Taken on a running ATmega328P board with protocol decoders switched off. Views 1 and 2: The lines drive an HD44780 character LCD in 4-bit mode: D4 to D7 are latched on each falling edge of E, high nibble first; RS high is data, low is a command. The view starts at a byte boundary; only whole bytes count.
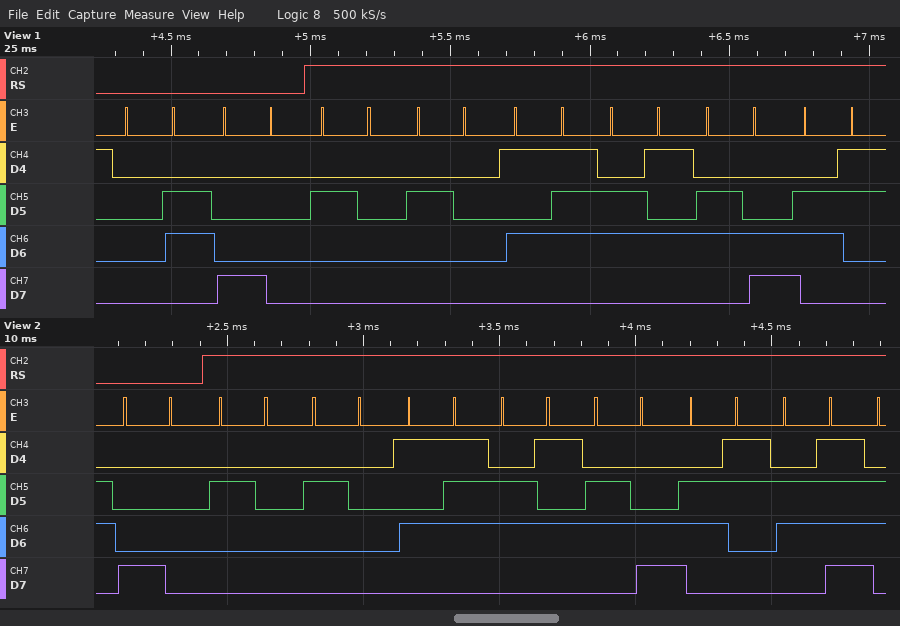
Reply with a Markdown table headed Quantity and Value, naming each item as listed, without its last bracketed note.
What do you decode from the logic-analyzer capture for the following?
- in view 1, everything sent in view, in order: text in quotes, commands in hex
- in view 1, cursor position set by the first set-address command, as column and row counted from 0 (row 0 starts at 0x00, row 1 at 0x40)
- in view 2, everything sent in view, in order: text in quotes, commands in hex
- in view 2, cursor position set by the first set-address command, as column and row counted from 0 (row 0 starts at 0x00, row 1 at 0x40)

| Quantity | Value |
|---|---|
| in view 1, everything sent in view, in order: text in quotes, commands in hex | 0x06 0x80 "  Welc" |
| in view 1, cursor position set by the first set-address command, as column and row counted from 0 | column 0, row 0 |
| in view 2, everything sent in view, in order: text in quotes, commands in hex | 0x80 "  Welco" |
| in view 2, cursor position set by the first set-address command, as column and row counted from 0 | column 0, row 0 |
